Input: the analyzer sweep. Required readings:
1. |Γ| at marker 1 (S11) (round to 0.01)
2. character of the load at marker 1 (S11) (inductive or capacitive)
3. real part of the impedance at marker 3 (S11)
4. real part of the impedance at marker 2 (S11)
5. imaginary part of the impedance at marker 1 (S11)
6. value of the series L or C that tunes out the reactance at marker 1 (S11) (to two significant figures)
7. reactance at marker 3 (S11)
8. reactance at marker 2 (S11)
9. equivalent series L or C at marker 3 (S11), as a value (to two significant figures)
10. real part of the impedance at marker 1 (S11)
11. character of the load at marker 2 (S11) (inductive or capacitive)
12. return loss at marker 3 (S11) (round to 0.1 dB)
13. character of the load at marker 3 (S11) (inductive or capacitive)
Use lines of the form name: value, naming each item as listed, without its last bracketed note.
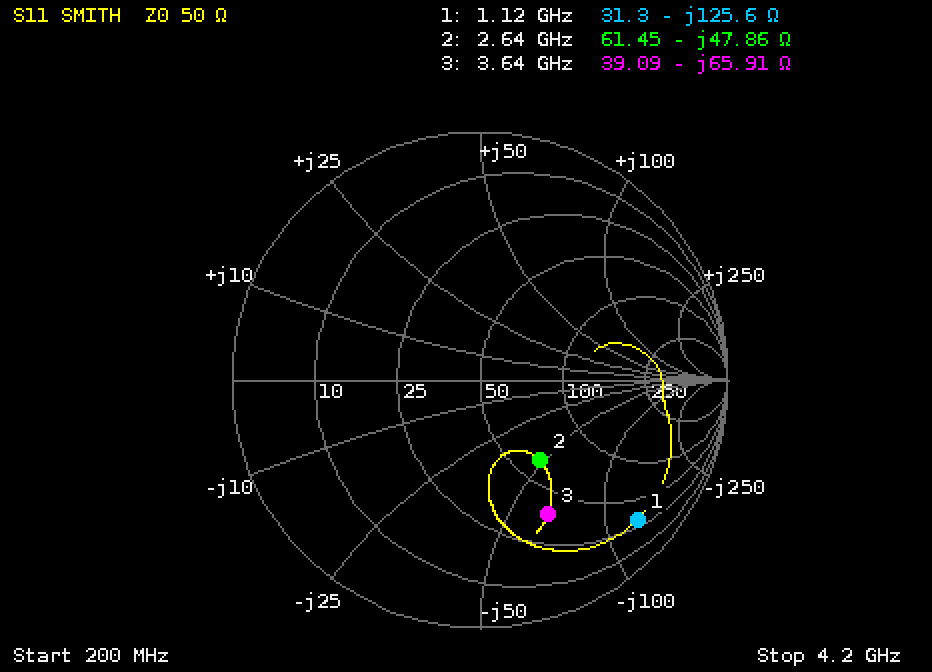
|Γ| at marker 1 (S11): 0.85
character of the load at marker 1 (S11): capacitive
real part of the impedance at marker 3: 39.09 Ω
real part of the impedance at marker 2: 61.45 Ω
imaginary part of the impedance at marker 1: -125.6 Ω
value of the series L or C that tunes out the reactance at marker 1 (S11): 18 nH
reactance at marker 3: -65.91 Ω
reactance at marker 2: -47.86 Ω
equivalent series L or C at marker 3 (S11), as a value: 660 fF
real part of the impedance at marker 1: 31.3 Ω
character of the load at marker 2 (S11): capacitive
return loss at marker 3 (S11): 4.4 dB
character of the load at marker 3 (S11): capacitive
